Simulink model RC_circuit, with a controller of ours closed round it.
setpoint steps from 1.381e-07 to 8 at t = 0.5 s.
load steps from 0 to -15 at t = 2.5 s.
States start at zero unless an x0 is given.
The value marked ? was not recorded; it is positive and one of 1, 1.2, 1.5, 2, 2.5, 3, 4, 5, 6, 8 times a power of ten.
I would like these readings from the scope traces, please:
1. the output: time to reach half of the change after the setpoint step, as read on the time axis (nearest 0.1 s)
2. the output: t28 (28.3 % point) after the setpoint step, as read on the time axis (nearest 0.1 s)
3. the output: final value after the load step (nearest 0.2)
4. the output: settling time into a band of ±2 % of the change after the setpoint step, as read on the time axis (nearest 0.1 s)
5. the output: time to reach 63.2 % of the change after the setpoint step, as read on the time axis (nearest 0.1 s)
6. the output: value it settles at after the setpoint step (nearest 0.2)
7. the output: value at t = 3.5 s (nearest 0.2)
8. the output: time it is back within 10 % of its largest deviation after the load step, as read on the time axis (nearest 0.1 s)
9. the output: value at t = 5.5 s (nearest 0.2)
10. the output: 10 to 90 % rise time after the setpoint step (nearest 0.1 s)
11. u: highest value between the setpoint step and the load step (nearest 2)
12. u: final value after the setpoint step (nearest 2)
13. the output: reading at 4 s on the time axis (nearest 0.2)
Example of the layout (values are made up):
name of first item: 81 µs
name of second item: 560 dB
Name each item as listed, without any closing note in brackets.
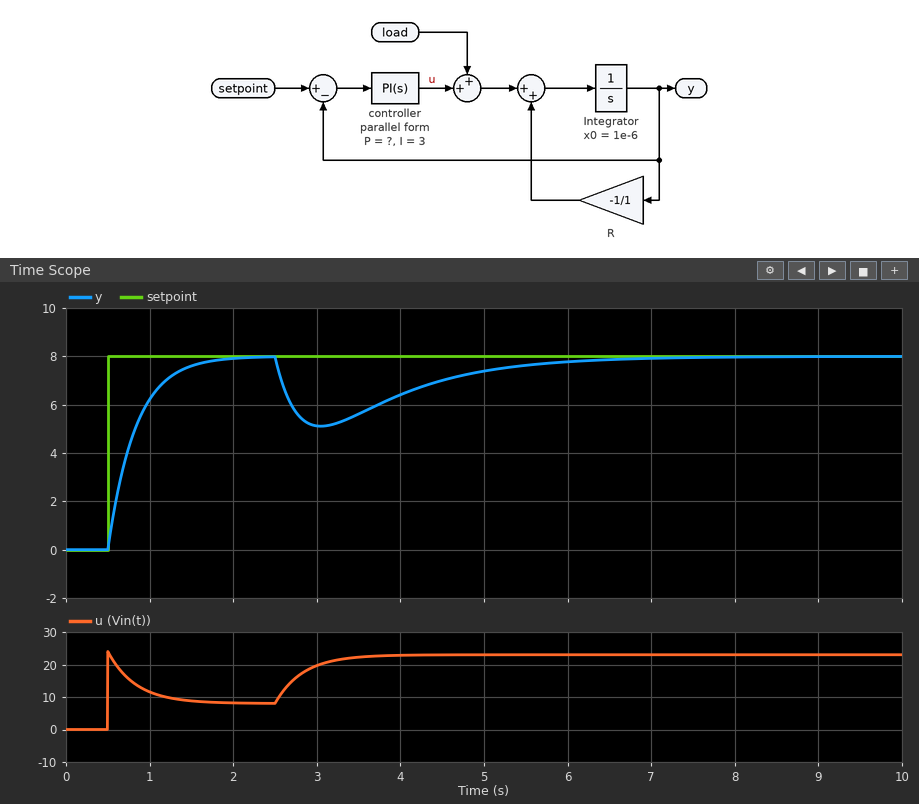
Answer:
the output: time to reach half of the change after the setpoint step, as read on the time axis: 0.7 s
the output: t28 (28.3 % point) after the setpoint step, as read on the time axis: 0.6 s
the output: final value after the load step: 8.0
the output: settling time into a band of ±2 % of the change after the setpoint step, as read on the time axis: 1.8 s
the output: time to reach 63.2 % of the change after the setpoint step, as read on the time axis: 0.8 s
the output: value it settles at after the setpoint step: 8.0
the output: value at t = 3.5 s: 5.6
the output: time it is back within 10 % of its largest deviation after the load step, as read on the time axis: 5.8 s
the output: value at t = 5.5 s: 7.6
the output: 10 to 90 % rise time after the setpoint step: 0.7 s
u: highest value between the setpoint step and the load step: 24
u: final value after the setpoint step: 8
the output: reading at 4 s on the time axis: 6.4
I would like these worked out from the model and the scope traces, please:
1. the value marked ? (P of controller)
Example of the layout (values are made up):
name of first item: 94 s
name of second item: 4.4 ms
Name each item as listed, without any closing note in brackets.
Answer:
the value marked ?: 3
